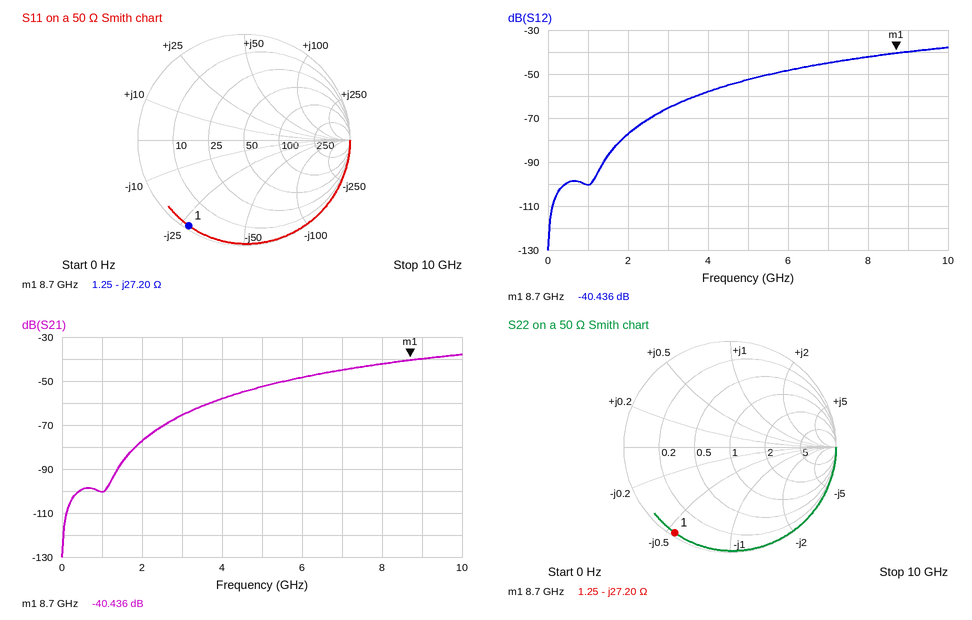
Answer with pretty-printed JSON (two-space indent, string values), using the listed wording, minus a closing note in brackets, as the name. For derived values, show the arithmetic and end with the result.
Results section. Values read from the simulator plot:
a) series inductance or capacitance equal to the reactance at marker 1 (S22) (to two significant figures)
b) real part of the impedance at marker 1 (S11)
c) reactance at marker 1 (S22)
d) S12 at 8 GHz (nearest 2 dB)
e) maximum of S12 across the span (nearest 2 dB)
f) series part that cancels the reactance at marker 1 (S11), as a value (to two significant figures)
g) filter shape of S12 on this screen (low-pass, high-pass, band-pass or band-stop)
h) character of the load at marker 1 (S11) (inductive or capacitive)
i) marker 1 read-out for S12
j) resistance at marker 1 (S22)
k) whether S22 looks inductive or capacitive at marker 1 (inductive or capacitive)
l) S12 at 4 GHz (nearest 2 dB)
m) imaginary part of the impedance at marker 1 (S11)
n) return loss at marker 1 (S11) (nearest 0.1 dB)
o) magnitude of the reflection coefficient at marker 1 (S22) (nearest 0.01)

{
  "series inductance or capacitance equal to the reactance at marker 1 (S22)": "C = 1/(2π × 8.7 GHz × 27.2 Ω) ≈ 673 fF, so 670 fF to two significant figures",
  "real part of the impedance at marker 1": "1.25 Ω",
  "reactance at marker 1": "-27.20 Ω",
  "S12 at 8 GHz": "-42 dB",
  "maximum of S12 across the span": "-38 dB",
  "series part that cancels the reactance at marker 1 (S11), as a value": "L = 27.2 Ω/(2π × 8.7 GHz) ≈ 498 pH, so 500 pH to two significant figures",
  "filter shape of S12 on this screen": "high-pass",
  "character of the load at marker 1 (S11)": "capacitive",
  "marker 1 read-out for S12": "-40.436 dB",
  "resistance at marker 1": "1.25 Ω",
  "whether S22 looks inductive or capacitive at marker 1": "capacitive",
  "S12 at 4 GHz": "-58 dB",
  "imaginary part of the impedance at marker 1": "-27.20 Ω",
  "return loss at marker 1 (S11)": "0.3 dB",
  "magnitude of the reflection coefficient at marker 1 (S22)": "0.96"
}
